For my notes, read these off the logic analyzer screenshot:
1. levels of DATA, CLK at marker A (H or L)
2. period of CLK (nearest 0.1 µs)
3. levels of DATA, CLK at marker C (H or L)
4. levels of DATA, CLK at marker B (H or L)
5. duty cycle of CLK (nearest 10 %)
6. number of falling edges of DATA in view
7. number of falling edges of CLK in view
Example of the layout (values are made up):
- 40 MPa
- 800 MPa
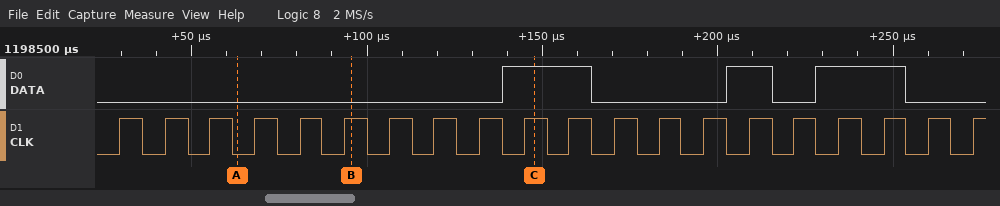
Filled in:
- DATA=L, CLK=L
- 12.8 µs
- DATA=H, CLK=H
- DATA=L, CLK=H
- 50 %
- 3
- 19
